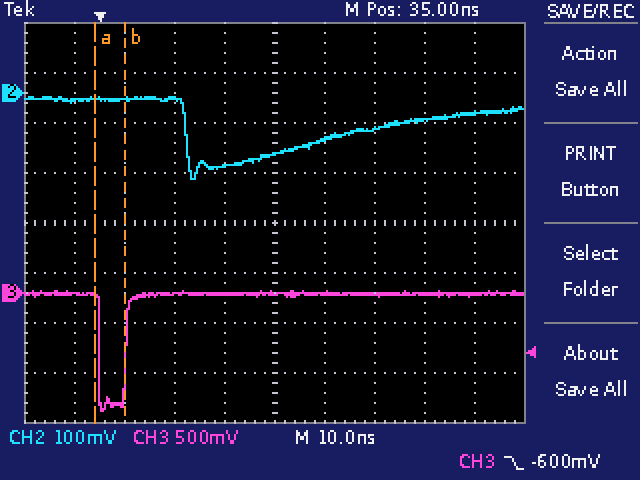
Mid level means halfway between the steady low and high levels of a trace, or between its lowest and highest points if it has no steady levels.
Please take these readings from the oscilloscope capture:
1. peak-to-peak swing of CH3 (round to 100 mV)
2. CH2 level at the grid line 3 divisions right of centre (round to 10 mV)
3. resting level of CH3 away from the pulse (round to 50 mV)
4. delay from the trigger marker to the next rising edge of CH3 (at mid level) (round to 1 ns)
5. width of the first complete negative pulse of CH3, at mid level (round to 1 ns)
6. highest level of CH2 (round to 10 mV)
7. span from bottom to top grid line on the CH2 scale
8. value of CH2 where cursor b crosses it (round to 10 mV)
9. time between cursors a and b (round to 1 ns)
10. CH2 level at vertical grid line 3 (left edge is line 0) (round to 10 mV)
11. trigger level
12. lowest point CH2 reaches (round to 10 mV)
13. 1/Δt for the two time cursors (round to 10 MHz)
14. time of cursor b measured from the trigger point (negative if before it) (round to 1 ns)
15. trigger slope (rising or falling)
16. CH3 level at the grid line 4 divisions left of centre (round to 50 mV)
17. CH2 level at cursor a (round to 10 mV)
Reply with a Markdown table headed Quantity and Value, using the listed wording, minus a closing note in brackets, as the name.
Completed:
| Quantity | Value |
|---|---|
| peak-to-peak swing of CH3 | 1.20 V |
| CH2 level at the grid line 3 divisions right of centre | -50 mV |
| resting level of CH3 away from the pulse | 0 mV |
| delay from the trigger marker to the next rising edge of CH3 (at mid level) | 5 ns |
| width of the first complete negative pulse of CH3, at mid level | 5 ns |
| highest level of CH2 | -10 mV |
| span from bottom to top grid line on the CH2 scale | 800 mV |
| value of CH2 where cursor b crosses it | -10 mV |
| time between cursors a and b | 6 ns |
| CH2 level at vertical grid line 3 (left edge is line 0) | -10 mV |
| trigger level | -600 mV |
| lowest point CH2 reaches | -170 mV |
| 1/Δt for the two time cursors | 170 MHz |
| time of cursor b measured from the trigger point (negative if before it) | +5 ns |
| trigger slope | falling |
| CH3 level at the grid line 4 divisions left of centre | 0 mV |
| CH2 level at cursor a | -10 mV |
